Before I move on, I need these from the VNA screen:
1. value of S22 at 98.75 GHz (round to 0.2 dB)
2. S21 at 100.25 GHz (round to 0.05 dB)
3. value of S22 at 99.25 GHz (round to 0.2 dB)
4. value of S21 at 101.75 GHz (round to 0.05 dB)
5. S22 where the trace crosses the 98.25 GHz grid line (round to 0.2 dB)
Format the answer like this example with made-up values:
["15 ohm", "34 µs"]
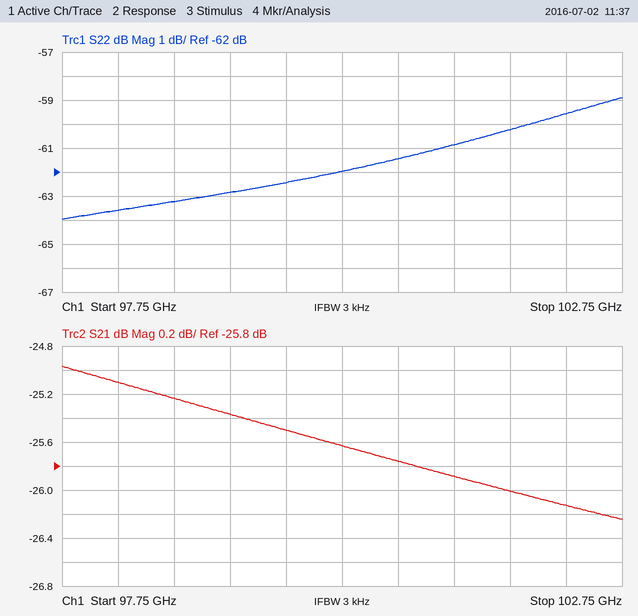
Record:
["-63.2 dB", "-25.65 dB", "-62.8 dB", "-26.00 dB", "-63.6 dB"]
